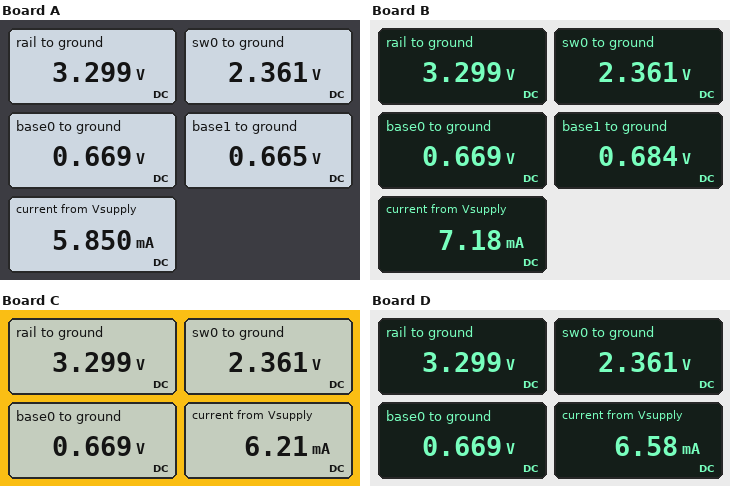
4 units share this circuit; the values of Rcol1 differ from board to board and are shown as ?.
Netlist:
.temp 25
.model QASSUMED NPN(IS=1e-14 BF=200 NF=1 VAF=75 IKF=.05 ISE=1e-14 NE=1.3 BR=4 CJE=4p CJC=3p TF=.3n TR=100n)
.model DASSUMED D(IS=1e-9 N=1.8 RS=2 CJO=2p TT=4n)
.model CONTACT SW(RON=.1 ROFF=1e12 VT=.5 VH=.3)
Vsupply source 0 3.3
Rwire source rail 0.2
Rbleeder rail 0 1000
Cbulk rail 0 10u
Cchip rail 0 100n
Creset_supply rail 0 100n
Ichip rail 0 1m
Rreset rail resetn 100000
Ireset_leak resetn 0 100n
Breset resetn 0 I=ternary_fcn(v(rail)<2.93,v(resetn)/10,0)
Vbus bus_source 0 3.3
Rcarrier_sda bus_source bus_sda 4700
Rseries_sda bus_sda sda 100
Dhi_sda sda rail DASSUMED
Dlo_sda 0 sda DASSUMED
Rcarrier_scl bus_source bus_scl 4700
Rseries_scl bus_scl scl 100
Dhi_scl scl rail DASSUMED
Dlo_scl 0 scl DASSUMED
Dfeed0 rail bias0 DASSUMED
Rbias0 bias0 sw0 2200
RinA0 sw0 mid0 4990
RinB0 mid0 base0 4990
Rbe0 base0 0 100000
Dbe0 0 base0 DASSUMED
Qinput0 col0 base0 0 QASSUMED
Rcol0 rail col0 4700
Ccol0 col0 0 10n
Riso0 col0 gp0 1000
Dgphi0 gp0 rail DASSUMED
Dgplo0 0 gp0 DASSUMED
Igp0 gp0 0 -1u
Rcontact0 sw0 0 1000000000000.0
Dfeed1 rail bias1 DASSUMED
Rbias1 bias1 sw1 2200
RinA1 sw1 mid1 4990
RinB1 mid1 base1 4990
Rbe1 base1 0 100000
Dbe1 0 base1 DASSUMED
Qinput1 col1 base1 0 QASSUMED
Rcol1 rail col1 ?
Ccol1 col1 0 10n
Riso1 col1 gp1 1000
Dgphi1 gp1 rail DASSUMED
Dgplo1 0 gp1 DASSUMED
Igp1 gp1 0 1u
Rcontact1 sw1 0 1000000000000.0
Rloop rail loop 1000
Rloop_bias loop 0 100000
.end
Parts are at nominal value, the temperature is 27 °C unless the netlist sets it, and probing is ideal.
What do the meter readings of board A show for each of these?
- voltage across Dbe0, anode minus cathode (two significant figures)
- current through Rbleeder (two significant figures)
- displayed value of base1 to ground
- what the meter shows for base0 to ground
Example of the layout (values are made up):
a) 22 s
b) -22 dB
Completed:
a) -670 mV
b) 3.3 mA
c) 0.665 V
d) 0.669 V
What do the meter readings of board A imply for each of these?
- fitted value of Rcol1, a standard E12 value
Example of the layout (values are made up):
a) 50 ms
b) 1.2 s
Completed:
a) 6.8 kΩ
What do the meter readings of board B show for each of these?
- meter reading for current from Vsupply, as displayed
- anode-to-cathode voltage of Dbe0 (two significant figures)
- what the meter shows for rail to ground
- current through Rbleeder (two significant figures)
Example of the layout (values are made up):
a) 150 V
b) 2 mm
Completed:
a) 7.18 mA
b) -670 mV
c) 3.299 V
d) 3.3 mA
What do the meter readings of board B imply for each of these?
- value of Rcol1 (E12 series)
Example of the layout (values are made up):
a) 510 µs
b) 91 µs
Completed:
a) 1.8 kΩ
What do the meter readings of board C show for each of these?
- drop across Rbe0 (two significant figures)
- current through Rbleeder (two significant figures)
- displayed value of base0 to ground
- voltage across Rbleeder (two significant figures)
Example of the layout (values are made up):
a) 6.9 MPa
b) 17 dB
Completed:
a) 670 mV
b) 3.3 mA
c) 0.669 V
d) 3.3 V
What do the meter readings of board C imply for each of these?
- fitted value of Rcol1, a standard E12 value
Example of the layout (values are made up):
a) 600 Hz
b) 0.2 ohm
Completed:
a) 3.9 kΩ
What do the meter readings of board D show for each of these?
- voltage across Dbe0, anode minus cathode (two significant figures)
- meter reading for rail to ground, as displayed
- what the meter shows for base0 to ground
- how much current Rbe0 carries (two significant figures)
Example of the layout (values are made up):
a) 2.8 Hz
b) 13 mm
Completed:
a) -670 mV
b) 3.299 V
c) 0.669 V
d) 6.7 µA
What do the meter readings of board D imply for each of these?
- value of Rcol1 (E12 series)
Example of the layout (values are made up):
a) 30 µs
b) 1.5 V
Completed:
a) 2.7 kΩ
